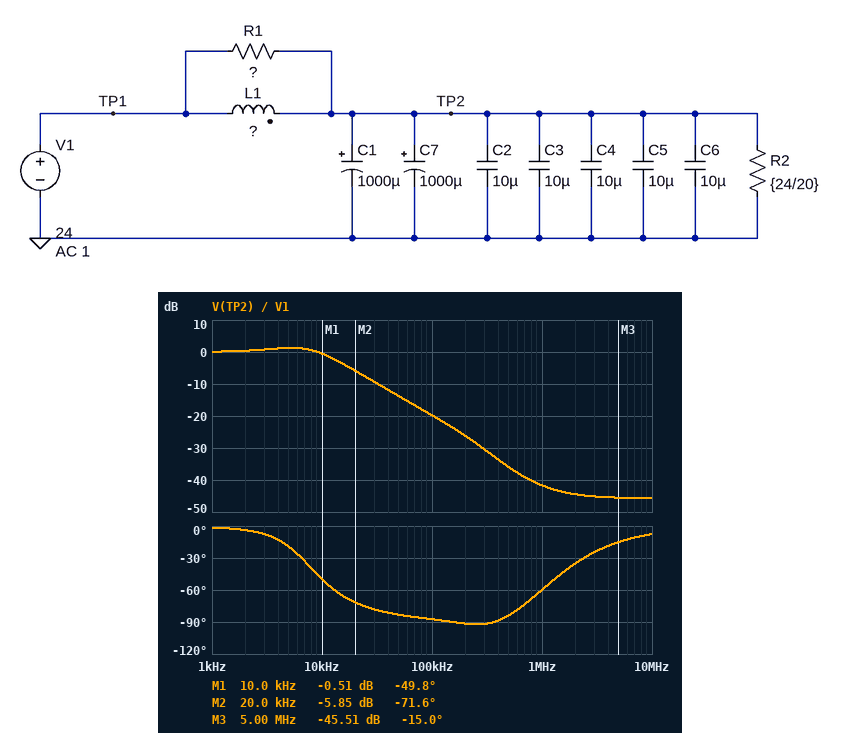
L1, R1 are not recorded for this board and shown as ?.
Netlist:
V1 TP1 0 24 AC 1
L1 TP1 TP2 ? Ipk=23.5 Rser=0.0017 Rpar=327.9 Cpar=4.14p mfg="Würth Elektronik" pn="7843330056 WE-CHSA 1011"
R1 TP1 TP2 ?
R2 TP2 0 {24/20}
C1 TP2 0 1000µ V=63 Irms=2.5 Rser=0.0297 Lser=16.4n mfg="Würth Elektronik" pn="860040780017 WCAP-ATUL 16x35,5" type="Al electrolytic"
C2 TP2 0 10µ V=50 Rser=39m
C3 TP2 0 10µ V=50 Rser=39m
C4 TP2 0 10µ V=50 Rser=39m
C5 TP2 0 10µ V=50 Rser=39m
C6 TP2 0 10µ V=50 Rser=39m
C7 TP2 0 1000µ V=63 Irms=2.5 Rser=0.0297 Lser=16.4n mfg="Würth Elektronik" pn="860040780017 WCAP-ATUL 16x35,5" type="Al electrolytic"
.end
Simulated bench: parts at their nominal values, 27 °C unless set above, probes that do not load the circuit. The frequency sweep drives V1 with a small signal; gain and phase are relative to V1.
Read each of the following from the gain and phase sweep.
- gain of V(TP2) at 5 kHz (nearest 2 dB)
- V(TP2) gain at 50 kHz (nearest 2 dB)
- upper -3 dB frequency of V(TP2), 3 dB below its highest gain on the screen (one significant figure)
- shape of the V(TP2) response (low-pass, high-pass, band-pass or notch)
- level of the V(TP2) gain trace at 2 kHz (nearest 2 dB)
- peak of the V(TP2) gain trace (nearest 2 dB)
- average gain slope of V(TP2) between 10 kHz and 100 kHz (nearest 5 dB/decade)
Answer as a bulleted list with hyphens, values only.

- 2 dB
- -14 dB
- 10 kHz
- low-pass
- 0 dB
- 2 dB
- -20 dB/decade
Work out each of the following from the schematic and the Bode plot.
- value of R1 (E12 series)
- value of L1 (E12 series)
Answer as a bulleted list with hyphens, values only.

- 1.5 Ω
- 220 nH
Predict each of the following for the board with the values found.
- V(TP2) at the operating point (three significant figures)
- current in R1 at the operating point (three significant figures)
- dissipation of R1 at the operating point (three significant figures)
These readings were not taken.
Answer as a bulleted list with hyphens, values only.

- 24.0 V
- 22.6 mA
- 767 µW
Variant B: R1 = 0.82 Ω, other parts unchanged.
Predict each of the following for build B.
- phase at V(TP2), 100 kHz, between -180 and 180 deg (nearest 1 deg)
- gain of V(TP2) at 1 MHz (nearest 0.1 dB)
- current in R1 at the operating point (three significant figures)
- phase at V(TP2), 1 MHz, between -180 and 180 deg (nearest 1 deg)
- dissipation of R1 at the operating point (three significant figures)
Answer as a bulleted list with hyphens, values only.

- -83 deg
- -38.5 dB
- 41.3 mA
- -43 deg
- 1.40 mW
